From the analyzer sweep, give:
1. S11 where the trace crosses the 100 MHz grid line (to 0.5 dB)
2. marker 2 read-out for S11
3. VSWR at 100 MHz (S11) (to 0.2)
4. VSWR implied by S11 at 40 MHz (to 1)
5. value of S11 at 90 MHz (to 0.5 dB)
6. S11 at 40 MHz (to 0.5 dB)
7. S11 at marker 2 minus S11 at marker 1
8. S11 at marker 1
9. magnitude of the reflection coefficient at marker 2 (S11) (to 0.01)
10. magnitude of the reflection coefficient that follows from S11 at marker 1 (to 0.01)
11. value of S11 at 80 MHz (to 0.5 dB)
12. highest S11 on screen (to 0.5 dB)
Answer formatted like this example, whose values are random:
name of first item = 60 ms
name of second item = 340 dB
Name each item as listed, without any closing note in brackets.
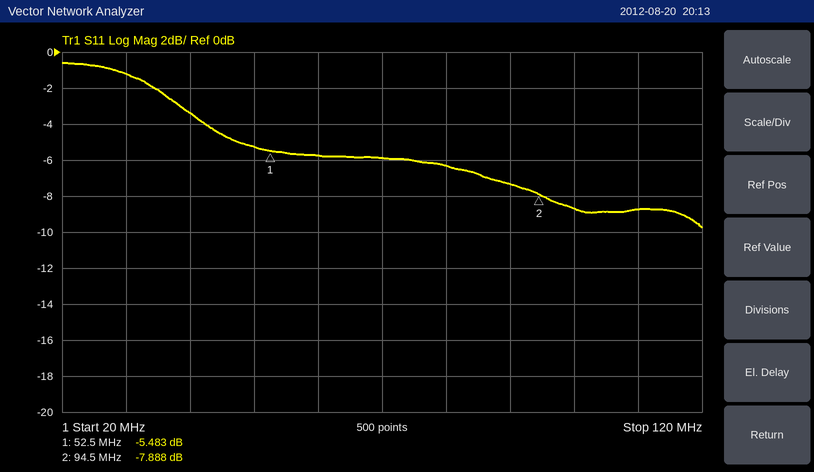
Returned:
S11 where the trace crosses the 100 MHz grid line = -8.5 dB
marker 2 read-out for S11 = -7.888 dB
VSWR at 100 MHz (S11) = 2.2
VSWR implied by S11 at 40 MHz = 5
value of S11 at 90 MHz = -7.5 dB
S11 at 40 MHz = -3.5 dB
S11 at marker 2 minus S11 at marker 1 = -2.405 dB
S11 at marker 1 = -5.483 dB
magnitude of the reflection coefficient at marker 2 (S11) = 0.40
magnitude of the reflection coefficient that follows from S11 at marker 1 = 0.53
value of S11 at 80 MHz = -6.5 dB
highest S11 on screen = -0.5 dB
